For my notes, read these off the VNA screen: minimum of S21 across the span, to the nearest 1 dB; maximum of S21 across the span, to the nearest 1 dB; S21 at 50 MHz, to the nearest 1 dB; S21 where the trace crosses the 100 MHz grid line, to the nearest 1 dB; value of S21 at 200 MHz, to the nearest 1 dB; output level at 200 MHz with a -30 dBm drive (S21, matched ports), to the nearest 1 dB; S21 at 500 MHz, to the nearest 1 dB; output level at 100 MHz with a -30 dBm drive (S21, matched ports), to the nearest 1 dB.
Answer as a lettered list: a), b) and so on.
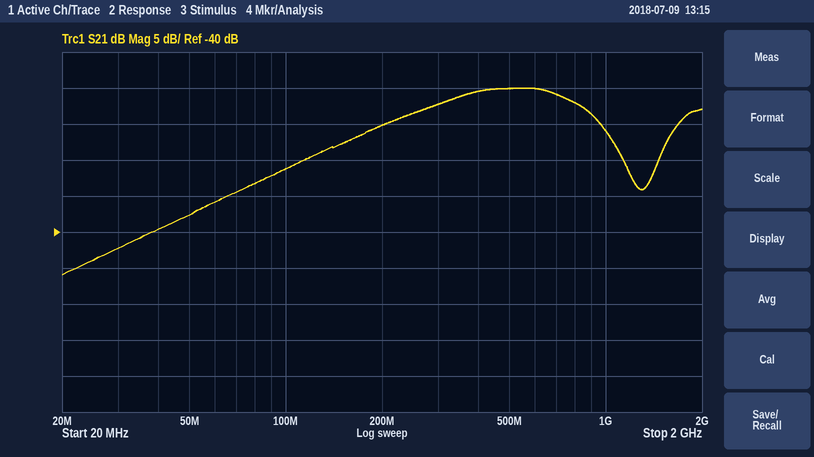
a) -46 dB
b) -20 dB
c) -38 dB
d) -31 dB
e) -25 dB
f) -55 dBm
g) -20 dB
h) -61 dBm
